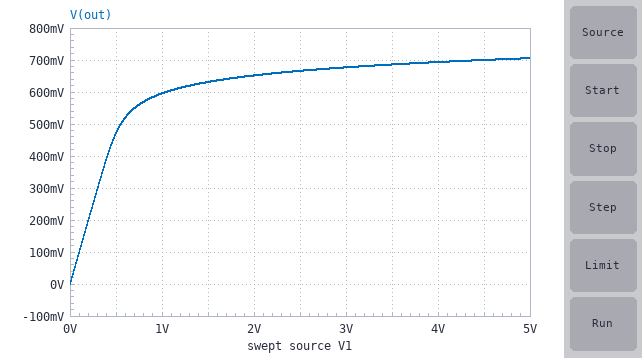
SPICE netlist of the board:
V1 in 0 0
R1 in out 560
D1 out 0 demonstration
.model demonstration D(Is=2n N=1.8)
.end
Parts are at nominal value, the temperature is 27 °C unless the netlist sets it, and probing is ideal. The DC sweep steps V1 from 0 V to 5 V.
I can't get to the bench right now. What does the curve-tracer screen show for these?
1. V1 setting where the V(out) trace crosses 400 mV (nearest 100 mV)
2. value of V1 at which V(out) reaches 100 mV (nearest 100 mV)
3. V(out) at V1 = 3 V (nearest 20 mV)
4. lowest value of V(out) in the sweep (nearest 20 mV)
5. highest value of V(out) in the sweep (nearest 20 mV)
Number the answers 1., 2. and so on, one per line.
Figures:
1. 400 mV
2. 100 mV
3. 680 mV
4. 0 V
5. 700 mV
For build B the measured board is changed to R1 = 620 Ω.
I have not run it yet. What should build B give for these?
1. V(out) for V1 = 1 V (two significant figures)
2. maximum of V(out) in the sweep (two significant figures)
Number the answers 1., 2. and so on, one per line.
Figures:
1. 590 mV
2. 700 mV
